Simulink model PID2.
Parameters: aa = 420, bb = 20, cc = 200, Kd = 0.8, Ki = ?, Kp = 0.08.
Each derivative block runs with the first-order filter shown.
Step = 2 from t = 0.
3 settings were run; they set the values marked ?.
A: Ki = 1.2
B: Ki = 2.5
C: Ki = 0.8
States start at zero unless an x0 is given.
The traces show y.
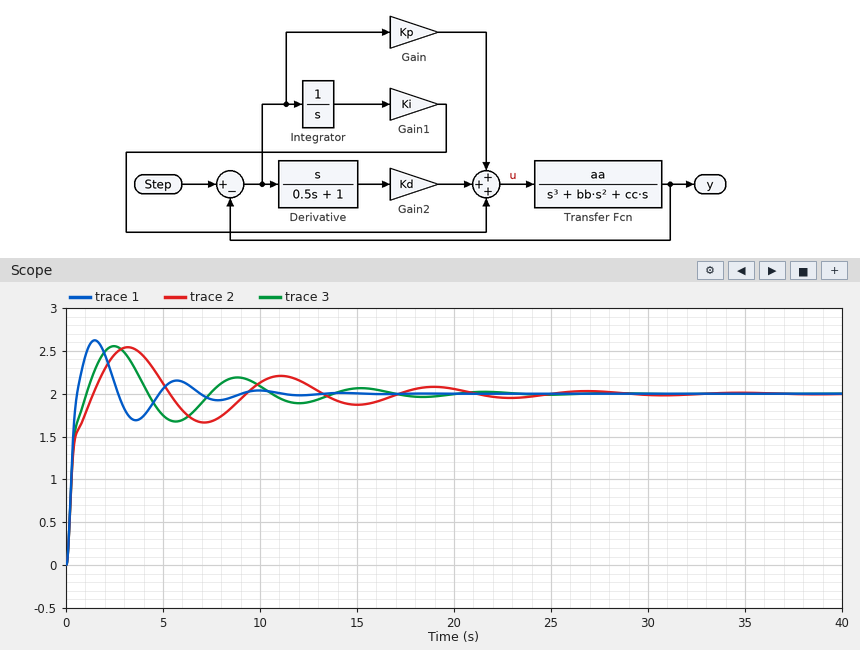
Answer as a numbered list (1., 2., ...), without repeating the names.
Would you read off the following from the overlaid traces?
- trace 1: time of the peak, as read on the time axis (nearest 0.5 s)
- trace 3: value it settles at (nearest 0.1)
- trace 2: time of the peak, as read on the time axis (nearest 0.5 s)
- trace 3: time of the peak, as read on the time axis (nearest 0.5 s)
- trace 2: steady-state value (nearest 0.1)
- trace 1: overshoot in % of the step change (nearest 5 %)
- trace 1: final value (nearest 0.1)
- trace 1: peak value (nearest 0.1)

1. 1.5 s
2. 2.0
3. 3.0 s
4. 2.5 s
5. 2.0
6. 30 %
7. 2.0
8. 2.6
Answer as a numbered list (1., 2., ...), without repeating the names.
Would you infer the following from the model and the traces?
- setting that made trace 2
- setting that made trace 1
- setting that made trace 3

1. C
2. B
3. A
